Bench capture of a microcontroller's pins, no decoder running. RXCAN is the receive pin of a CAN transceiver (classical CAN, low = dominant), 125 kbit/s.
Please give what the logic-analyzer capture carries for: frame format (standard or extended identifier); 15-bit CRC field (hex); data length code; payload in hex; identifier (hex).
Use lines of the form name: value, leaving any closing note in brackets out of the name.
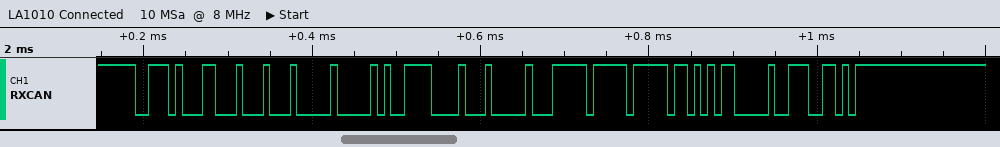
frame format: standard
15-bit CRC field: 0x00E6
data length code: 8
payload in hex: 88 00 9E 11 00 FF FF AB
identifier: 0x3A3
